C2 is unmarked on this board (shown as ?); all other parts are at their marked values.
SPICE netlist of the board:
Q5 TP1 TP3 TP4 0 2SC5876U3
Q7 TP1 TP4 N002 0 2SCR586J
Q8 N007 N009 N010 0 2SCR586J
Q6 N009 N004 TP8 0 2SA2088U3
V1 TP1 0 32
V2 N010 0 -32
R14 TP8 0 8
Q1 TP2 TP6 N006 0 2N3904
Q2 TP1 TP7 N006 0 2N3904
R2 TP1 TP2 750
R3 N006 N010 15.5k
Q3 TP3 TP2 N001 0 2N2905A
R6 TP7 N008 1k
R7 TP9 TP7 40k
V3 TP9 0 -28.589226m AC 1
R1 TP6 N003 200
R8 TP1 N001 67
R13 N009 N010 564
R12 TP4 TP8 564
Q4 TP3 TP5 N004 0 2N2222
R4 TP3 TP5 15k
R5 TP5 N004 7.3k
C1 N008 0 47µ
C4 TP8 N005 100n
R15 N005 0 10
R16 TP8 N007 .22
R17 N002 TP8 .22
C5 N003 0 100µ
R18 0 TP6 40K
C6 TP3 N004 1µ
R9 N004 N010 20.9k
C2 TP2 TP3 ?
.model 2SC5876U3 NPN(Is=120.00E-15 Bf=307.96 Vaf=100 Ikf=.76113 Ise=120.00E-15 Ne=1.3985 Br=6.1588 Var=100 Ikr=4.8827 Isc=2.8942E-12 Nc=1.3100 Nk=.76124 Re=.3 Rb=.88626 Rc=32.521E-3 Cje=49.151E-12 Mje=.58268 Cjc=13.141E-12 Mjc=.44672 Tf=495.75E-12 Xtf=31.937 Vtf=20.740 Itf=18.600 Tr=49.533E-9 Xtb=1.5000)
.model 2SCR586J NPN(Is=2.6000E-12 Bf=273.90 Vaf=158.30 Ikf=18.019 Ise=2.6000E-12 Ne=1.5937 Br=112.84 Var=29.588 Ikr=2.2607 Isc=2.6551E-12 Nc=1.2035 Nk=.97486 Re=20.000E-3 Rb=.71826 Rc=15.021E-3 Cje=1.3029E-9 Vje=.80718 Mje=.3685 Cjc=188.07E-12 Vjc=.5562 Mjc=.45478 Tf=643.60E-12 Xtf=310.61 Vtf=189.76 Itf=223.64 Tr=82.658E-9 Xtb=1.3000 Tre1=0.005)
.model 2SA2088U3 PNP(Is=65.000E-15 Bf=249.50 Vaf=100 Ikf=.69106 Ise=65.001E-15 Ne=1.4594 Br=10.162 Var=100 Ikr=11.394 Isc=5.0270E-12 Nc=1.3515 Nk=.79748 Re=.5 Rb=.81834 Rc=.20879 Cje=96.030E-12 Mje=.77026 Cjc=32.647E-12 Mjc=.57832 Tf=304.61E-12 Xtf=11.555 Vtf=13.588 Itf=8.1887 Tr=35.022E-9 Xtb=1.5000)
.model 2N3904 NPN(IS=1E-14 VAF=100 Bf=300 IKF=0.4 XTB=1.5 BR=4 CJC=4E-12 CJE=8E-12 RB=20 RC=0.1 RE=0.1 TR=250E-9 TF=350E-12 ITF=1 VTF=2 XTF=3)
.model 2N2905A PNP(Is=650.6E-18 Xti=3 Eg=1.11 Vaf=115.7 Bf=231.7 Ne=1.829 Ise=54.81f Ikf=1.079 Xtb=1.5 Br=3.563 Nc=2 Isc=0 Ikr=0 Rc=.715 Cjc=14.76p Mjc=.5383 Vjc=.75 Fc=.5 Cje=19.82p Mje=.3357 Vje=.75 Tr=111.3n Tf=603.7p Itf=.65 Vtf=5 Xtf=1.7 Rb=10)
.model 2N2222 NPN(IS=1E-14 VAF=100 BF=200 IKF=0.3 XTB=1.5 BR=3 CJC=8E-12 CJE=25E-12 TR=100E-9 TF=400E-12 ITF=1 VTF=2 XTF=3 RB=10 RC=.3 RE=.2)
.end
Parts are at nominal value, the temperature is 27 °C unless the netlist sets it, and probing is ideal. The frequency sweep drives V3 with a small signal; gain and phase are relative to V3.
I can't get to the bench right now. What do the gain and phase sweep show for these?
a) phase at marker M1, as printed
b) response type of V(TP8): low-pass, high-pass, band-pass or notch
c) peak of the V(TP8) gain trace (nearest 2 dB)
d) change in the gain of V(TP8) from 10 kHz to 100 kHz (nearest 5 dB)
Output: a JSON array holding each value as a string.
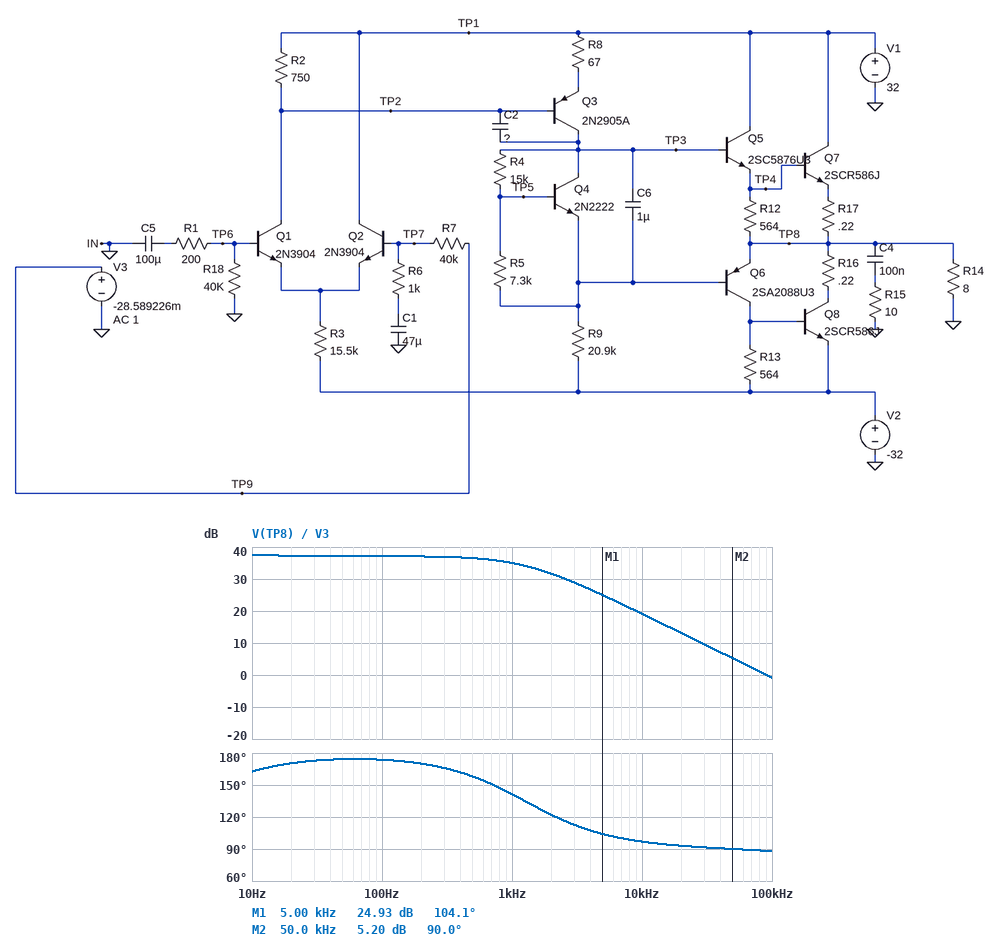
["104.1 deg", "low-pass", "38 dB", "-20 dB"]
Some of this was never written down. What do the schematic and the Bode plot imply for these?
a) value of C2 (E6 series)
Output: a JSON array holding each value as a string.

["680 pF"]
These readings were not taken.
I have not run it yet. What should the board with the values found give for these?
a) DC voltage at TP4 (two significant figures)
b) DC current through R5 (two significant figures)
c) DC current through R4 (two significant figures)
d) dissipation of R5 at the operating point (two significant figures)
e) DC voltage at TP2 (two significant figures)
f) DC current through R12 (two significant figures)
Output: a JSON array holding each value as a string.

["840 mV", "91 µA", "98 µA", "60 µW", "31 V", "1.5 mA"]
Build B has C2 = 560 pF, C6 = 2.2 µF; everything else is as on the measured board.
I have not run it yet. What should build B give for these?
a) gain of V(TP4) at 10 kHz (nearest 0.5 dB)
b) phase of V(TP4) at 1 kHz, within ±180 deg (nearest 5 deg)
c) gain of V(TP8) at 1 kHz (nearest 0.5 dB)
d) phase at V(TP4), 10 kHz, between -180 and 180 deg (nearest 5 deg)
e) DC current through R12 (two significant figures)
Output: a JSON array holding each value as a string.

["21.0 dB", "145 deg", "35.5 dB", "100 deg", "1.5 mA"]
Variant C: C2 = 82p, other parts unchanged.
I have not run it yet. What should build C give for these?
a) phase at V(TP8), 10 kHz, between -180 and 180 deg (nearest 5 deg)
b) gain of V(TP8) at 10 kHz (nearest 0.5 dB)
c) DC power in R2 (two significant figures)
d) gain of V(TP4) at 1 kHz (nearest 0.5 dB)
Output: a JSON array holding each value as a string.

["135 deg", "34.0 dB", "920 µW", "37.0 dB"]
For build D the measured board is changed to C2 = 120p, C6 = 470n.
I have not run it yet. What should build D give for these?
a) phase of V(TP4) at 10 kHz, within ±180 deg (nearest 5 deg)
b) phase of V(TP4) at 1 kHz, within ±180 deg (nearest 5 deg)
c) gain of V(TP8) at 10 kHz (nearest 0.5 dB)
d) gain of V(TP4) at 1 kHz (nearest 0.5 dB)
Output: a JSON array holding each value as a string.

["125 deg", "170 deg", "32.5 dB", "37.0 dB"]
